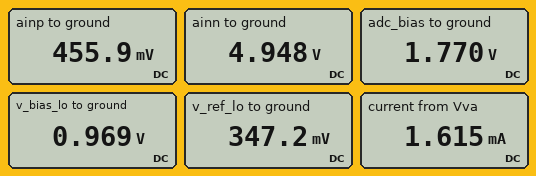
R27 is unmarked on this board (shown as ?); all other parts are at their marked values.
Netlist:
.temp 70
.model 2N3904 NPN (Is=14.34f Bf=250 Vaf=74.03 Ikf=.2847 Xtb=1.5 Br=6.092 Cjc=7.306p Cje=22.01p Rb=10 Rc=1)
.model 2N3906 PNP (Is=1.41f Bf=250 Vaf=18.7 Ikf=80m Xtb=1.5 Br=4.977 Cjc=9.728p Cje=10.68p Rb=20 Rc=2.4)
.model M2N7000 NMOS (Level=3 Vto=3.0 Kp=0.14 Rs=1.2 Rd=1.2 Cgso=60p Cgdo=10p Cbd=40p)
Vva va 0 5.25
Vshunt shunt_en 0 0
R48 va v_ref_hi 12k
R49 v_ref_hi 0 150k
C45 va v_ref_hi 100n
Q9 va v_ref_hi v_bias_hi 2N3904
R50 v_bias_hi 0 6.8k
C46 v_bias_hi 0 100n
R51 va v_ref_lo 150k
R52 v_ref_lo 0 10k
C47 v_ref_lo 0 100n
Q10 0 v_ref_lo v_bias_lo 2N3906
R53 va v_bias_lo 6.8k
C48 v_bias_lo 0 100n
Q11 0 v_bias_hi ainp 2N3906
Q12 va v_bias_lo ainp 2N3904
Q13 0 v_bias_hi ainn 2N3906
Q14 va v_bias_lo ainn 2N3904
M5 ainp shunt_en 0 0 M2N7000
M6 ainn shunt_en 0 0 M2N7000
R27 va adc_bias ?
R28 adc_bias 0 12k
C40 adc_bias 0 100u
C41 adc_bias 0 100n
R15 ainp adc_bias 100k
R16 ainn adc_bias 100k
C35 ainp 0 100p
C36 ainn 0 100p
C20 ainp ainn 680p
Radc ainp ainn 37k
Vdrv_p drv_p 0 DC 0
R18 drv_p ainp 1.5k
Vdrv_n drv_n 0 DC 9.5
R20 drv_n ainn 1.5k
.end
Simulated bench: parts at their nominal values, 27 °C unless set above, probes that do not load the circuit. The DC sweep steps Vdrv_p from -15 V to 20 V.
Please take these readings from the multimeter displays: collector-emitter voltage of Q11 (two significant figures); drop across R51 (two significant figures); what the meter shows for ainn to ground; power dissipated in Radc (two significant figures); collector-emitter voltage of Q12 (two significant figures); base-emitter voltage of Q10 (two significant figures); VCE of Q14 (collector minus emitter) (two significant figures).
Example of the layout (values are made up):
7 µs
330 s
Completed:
-460 mV
4.9 V
4.948 V
550 µW
4.8 V
-620 mV
300 mV
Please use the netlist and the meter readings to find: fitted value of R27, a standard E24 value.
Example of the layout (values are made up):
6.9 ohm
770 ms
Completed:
27 kΩ
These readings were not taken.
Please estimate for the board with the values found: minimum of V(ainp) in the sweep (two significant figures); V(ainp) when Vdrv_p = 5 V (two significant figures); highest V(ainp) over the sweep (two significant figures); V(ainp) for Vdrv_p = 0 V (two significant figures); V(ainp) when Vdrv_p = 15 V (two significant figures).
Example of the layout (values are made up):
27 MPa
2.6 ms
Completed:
330 mV
4.8 V
5.0 V
460 mV
5.0 V
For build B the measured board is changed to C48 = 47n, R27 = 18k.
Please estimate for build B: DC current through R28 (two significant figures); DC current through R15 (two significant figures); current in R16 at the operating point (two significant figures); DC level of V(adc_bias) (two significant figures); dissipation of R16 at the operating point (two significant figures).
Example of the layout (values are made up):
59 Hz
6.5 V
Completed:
180 µA
17 µA
28 µA
2.2 V
77 µW
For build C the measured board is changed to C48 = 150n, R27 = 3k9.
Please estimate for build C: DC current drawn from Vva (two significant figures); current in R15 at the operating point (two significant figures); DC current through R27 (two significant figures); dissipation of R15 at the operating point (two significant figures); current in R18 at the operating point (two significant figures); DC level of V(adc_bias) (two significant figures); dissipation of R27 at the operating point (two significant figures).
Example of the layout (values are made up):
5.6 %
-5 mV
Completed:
1.8 mA
34 µA
350 µA
120 µW
310 µA
3.9 V
470 µW
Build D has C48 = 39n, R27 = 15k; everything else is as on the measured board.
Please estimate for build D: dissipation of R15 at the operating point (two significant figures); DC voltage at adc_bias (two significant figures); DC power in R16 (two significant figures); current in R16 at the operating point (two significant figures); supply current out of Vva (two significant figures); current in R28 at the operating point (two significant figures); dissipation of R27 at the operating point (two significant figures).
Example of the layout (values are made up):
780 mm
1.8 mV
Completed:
37 µW
2.4 V
66 µW
26 µA
1.7 mA
200 µA
550 µW
